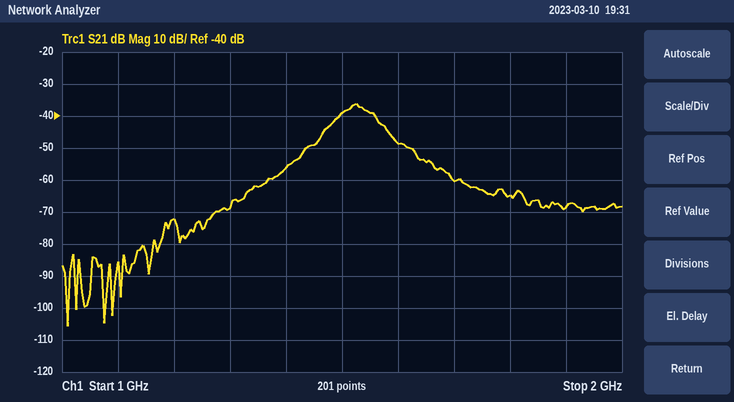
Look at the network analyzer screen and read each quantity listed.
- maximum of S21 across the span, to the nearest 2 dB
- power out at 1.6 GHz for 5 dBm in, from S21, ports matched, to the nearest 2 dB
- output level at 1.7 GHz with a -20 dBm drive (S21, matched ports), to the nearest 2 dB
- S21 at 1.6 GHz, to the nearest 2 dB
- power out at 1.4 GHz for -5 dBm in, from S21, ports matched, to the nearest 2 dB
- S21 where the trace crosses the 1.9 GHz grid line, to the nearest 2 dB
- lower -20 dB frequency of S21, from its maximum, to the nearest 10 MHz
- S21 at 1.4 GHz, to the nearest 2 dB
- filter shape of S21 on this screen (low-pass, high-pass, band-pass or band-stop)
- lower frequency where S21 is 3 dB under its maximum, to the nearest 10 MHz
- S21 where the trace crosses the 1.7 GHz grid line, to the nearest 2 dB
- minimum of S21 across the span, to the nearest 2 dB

-36 dB
-44 dBm
-80 dBm
-48 dB
-62 dBm
-68 dB
1.40 GHz
-56 dB
band-pass
1.50 GHz
-60 dB
-106 dB
